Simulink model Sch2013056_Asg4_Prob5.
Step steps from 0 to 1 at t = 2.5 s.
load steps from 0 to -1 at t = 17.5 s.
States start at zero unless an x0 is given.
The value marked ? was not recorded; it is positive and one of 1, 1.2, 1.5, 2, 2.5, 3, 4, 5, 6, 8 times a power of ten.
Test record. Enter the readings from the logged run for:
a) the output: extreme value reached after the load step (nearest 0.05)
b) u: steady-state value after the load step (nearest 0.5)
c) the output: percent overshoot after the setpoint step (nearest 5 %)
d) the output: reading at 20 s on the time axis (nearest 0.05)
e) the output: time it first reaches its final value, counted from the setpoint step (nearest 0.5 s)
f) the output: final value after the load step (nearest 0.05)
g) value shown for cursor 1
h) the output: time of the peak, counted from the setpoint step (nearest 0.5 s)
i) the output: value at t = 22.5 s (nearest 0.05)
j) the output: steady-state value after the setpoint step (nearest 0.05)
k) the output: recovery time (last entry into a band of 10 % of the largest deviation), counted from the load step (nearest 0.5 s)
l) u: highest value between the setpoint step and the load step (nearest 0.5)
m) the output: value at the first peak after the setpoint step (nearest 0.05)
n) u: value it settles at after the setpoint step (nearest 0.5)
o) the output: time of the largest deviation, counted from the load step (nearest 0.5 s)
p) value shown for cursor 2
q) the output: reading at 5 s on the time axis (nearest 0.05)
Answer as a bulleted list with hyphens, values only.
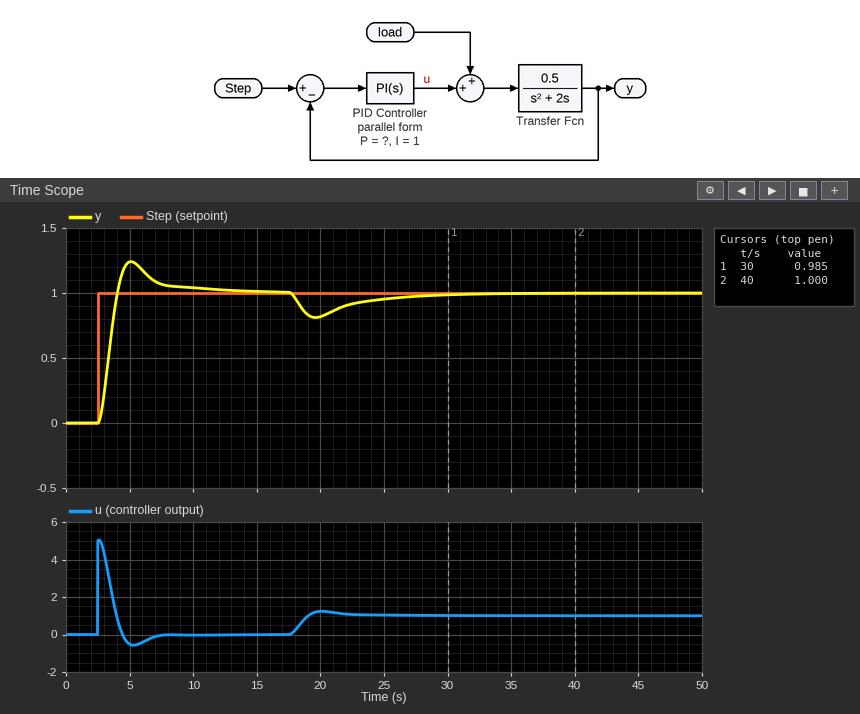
- 0.80
- 1.0
- 25 %
- 0.80
- 1.5 s
- 1.00
- 0.985
- 2.5 s
- 0.90
- 1.00
- 11.0 s
- 5.0
- 1.25
- 0.0
- 2.0 s
- 1.000
- 1.25
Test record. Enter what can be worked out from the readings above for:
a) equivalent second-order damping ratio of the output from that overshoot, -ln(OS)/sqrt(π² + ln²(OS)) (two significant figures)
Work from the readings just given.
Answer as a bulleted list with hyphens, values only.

- 0.40
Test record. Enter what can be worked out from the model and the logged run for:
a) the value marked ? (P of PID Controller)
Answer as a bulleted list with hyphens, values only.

- 5
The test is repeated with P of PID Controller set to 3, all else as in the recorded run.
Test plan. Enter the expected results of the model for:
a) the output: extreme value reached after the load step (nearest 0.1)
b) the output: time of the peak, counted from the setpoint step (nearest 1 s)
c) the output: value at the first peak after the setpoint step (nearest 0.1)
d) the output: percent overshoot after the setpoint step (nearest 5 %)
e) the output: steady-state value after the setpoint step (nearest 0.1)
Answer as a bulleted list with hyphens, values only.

- 0.7
- 4 s
- 1.3
- 35 %
- 1.0
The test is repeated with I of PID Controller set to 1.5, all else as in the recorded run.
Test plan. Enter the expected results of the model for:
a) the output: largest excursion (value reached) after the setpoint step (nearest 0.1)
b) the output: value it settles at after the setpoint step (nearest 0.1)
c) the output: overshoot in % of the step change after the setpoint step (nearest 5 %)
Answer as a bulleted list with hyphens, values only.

- 1.3
- 1.0
- 30 %
